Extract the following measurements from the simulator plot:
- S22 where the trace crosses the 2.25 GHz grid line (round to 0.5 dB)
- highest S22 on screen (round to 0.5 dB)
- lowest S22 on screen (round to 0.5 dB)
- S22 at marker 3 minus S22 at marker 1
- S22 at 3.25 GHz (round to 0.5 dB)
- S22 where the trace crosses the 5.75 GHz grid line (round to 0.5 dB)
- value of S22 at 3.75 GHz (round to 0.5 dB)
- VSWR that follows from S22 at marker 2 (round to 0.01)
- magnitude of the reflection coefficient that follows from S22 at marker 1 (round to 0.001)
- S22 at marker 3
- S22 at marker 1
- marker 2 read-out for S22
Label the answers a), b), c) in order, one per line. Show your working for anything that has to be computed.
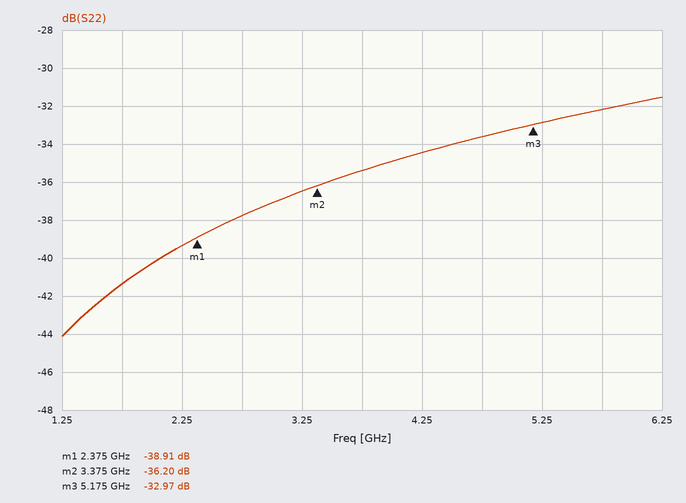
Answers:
a) -39.5 dB
b) -31.5 dB
c) -44.0 dB
d) -32.97 − (-38.91) = 5.94 dB
e) -36.5 dB
f) -32.0 dB
g) -35.5 dB
h) (1 + 0.0155)/(1 − 0.0155) ≈ 1.03
i) 10^(-38.91/20) ≈ 0.011
j) -32.97 dB
k) -38.91 dB
l) -36.20 dB
